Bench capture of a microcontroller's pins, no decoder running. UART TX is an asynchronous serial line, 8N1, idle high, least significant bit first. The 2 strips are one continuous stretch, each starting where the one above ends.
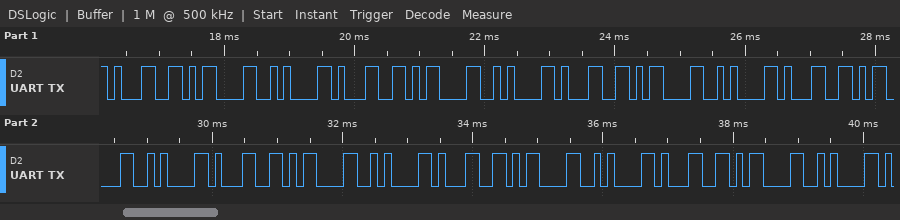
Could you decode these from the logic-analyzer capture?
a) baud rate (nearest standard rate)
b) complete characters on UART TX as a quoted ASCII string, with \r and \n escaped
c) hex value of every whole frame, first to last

9600 baud
"1\r\n1\r\n1\r\n1\r\n1\r\n1\r\n1\r\n"
31 0D 0A 31 0D 0A 31 0D 0A 31 0D 0A 31 0D 0A 31 0D 0A 31 0D 0A
